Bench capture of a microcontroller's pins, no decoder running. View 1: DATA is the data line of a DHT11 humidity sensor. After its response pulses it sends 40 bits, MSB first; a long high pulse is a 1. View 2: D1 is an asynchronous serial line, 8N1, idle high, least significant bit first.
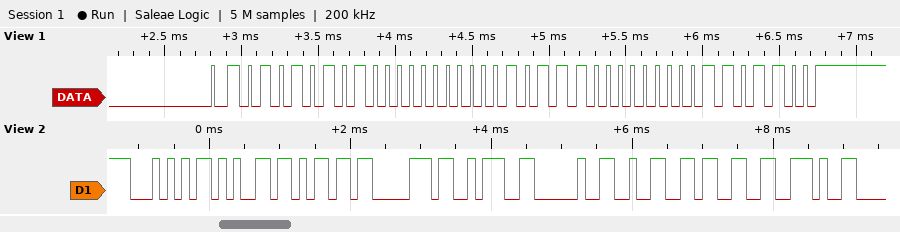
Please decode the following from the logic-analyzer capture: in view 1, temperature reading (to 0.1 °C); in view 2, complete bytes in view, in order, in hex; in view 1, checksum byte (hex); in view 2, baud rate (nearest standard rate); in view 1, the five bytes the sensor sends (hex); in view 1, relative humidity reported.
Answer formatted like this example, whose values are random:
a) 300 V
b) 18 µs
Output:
a) 23.0 °C
b) 54 65 6D 70 3A 20 32 33 2E
c) 0x6C
d) 9600 baud
e) 55 00 17 00 6C
f) 85 %
